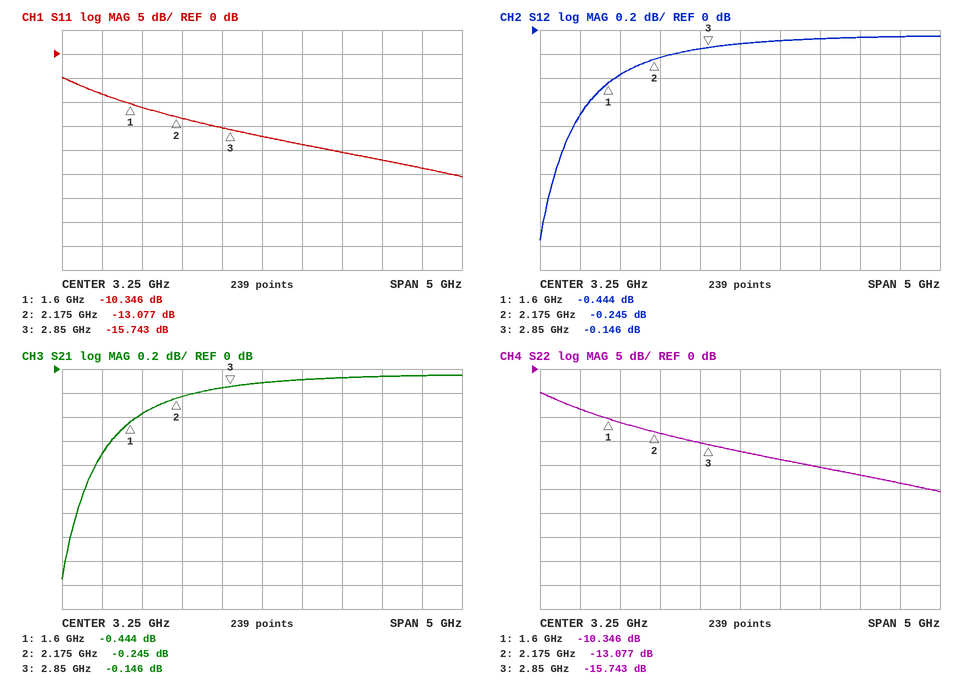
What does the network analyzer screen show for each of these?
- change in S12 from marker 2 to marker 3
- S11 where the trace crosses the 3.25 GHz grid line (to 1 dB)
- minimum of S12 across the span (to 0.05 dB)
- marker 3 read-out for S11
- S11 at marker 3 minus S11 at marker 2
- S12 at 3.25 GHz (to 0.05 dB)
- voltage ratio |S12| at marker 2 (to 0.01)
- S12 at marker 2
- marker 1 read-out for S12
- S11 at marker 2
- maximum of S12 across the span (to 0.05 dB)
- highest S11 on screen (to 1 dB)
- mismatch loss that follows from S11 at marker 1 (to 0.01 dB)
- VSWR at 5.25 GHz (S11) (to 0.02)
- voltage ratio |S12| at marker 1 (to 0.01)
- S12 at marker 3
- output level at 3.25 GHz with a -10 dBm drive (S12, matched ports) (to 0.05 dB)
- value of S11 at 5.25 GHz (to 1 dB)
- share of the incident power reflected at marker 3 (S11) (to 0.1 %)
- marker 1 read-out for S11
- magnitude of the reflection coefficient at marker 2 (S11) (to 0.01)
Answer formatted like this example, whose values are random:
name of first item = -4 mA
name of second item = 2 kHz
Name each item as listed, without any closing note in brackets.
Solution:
change in S12 from marker 2 to marker 3 = 0.099 dB
S11 where the trace crosses the 3.25 GHz grid line = -17 dB
minimum of S12 across the span = -1.75 dB
marker 3 read-out for S11 = -15.743 dB
S11 at marker 3 minus S11 at marker 2 = -2.666 dB
S12 at 3.25 GHz = -0.10 dB
voltage ratio |S12| at marker 2 = 0.97
S12 at marker 2 = -0.245 dB
marker 1 read-out for S12 = -0.444 dB
S11 at marker 2 = -13.077 dB
maximum of S12 across the span = -0.05 dB
highest S11 on screen = -5 dB
mismatch loss that follows from S11 at marker 1 = 0.42 dB
VSWR at 5.25 GHz (S11) = 1.14
voltage ratio |S12| at marker 1 = 0.95
S12 at marker 3 = -0.146 dB
output level at 3.25 GHz with a -10 dBm drive (S12, matched ports) = -10.10 dBm
value of S11 at 5.25 GHz = -24 dB
share of the incident power reflected at marker 3 (S11) = 2.7 %
marker 1 read-out for S11 = -10.346 dB
magnitude of the reflection coefficient at marker 2 (S11) = 0.22
